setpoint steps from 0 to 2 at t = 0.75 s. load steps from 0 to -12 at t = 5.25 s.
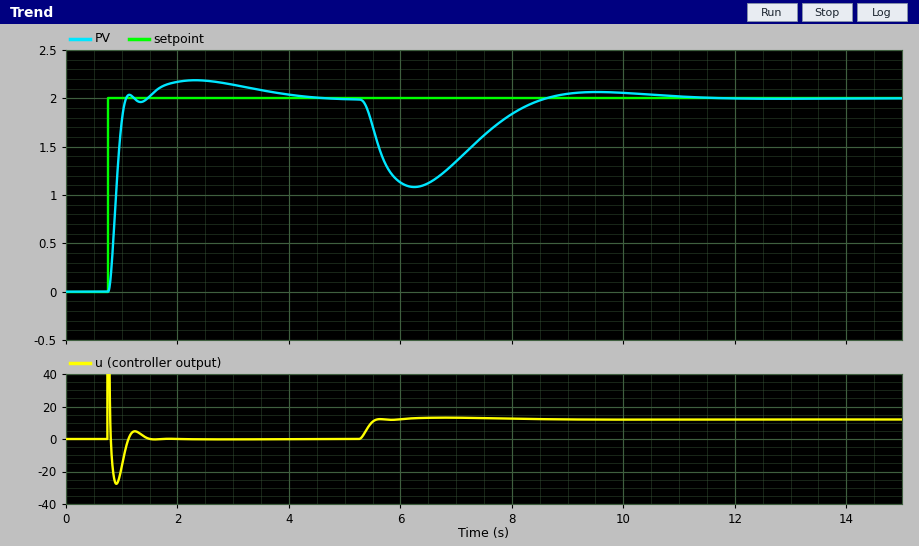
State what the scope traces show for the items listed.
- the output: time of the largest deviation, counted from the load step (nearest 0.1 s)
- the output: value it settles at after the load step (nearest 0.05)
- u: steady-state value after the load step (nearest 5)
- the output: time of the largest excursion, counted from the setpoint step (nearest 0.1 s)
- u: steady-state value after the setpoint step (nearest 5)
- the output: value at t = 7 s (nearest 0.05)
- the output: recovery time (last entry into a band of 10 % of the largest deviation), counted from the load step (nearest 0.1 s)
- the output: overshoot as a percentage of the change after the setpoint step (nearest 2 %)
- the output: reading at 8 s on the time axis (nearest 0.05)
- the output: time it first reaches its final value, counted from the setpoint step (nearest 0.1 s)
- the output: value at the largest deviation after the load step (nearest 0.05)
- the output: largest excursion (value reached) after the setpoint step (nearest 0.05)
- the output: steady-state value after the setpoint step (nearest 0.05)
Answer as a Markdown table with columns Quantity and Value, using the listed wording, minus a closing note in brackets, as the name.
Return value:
| Quantity | Value |
|---|---|
| the output: time of the largest deviation, counted from the load step | 1.0 s |
| the output: value it settles at after the load step | 2.00 |
| u: steady-state value after the load step | 10 |
| the output: time of the largest excursion, counted from the setpoint step | 1.6 s |
| u: steady-state value after the setpoint step | 0 |
| the output: value at t = 7 s | 1.35 |
| the output: recovery time (last entry into a band of 10 % of the largest deviation), counted from the load step | 3.0 s |
| the output: overshoot as a percentage of the change after the setpoint step | 10 % |
| the output: reading at 8 s on the time axis | 1.85 |
| the output: time it first reaches its final value, counted from the setpoint step | 0.3 s |
| the output: value at the largest deviation after the load step | 1.10 |
| the output: largest excursion (value reached) after the setpoint step | 2.20 |
| the output: steady-state value after the setpoint step | 2.00 |
